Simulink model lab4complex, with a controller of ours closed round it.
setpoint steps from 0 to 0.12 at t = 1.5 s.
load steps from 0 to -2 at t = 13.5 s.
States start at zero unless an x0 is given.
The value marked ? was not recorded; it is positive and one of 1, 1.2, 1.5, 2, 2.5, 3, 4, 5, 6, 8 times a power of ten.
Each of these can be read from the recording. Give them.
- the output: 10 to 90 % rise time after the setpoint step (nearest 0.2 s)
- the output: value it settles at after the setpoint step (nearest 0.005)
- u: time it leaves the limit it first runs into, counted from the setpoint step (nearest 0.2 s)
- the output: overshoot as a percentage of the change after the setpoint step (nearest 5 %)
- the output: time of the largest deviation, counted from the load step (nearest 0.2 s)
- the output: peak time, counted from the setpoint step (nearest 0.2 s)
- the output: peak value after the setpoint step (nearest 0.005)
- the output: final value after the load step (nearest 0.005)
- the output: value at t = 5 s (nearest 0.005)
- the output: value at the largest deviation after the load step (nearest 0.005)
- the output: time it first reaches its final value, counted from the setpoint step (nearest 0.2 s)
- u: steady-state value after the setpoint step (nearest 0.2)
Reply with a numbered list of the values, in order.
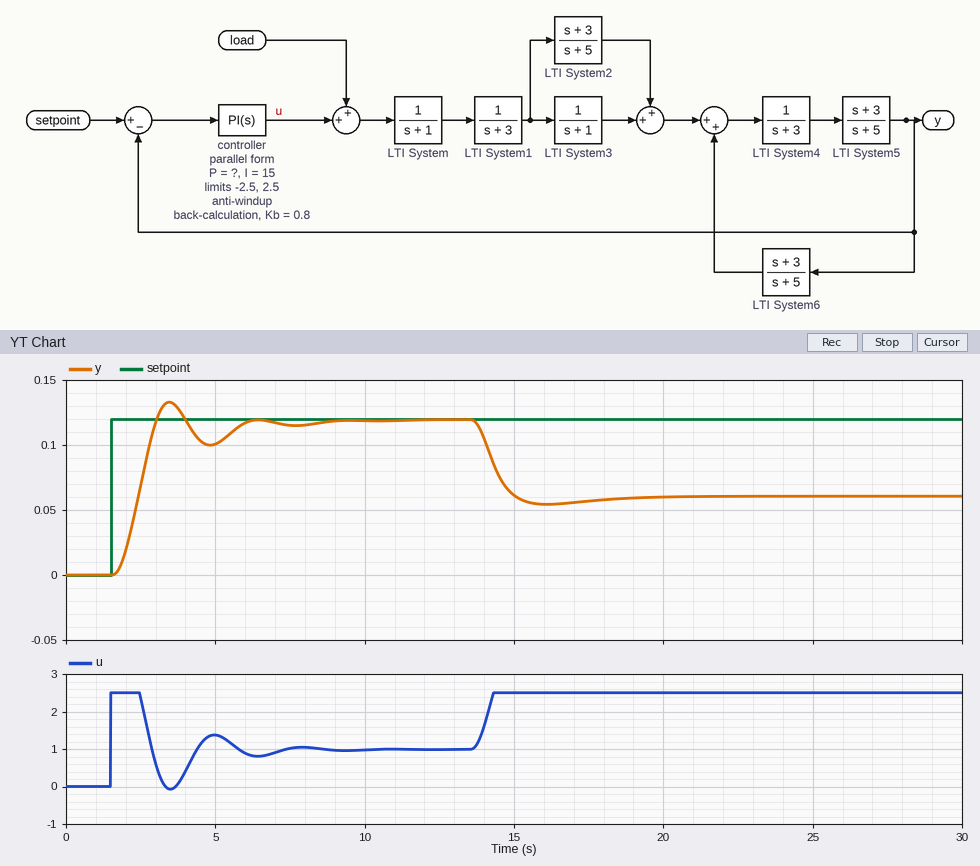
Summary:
1. 1.0 s
2. 0.120
3. 1.0 s
4. 10 %
5. 2.6 s
6. 2.0 s
7. 0.135
8. 0.060
9. 0.100
10. 0.055
11. 1.6 s
12. 1.0
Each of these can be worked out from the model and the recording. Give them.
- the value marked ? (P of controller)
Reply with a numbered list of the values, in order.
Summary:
1. 40
